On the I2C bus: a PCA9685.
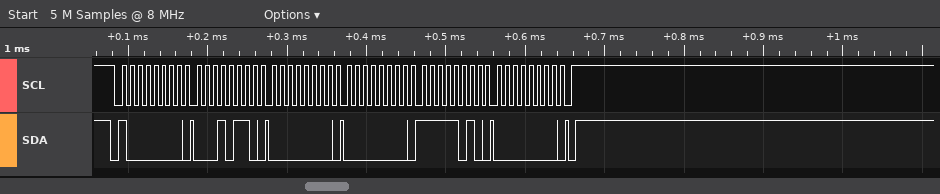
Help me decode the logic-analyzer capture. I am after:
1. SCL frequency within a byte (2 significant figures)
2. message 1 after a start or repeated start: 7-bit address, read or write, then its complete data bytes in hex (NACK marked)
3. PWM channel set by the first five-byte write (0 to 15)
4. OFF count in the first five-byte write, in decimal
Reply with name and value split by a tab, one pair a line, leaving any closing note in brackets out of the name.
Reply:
SCL frequency within a byte	100 kHz
message 1 after a start or repeated start: 7-bit address, read or write, then its complete data bytes in hex	0x40 write: 16 00 00 FA 00
PWM channel set by the first five-byte write	4
OFF count in the first five-byte write, in decimal	250
